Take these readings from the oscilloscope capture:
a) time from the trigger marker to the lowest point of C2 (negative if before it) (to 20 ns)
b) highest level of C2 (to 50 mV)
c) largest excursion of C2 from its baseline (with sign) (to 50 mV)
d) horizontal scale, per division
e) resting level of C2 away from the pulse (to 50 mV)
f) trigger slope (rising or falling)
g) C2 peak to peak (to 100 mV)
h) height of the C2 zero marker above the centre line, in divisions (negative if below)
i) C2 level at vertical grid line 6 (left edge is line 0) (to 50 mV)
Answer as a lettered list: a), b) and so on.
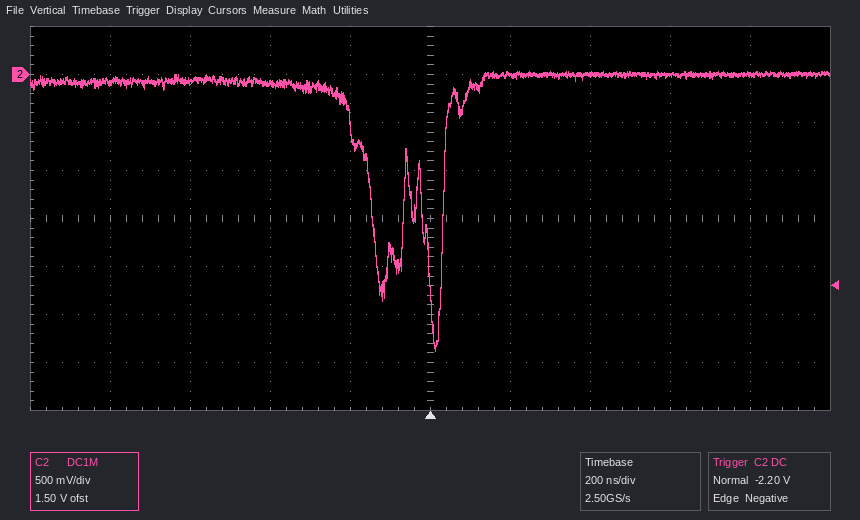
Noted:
a) +20 ns
b) 50 mV
c) -2.80 V
d) 200 ns
e) -50 mV
f) falling
g) 2.90 V
h) +3.0 div
i) 0 mV
